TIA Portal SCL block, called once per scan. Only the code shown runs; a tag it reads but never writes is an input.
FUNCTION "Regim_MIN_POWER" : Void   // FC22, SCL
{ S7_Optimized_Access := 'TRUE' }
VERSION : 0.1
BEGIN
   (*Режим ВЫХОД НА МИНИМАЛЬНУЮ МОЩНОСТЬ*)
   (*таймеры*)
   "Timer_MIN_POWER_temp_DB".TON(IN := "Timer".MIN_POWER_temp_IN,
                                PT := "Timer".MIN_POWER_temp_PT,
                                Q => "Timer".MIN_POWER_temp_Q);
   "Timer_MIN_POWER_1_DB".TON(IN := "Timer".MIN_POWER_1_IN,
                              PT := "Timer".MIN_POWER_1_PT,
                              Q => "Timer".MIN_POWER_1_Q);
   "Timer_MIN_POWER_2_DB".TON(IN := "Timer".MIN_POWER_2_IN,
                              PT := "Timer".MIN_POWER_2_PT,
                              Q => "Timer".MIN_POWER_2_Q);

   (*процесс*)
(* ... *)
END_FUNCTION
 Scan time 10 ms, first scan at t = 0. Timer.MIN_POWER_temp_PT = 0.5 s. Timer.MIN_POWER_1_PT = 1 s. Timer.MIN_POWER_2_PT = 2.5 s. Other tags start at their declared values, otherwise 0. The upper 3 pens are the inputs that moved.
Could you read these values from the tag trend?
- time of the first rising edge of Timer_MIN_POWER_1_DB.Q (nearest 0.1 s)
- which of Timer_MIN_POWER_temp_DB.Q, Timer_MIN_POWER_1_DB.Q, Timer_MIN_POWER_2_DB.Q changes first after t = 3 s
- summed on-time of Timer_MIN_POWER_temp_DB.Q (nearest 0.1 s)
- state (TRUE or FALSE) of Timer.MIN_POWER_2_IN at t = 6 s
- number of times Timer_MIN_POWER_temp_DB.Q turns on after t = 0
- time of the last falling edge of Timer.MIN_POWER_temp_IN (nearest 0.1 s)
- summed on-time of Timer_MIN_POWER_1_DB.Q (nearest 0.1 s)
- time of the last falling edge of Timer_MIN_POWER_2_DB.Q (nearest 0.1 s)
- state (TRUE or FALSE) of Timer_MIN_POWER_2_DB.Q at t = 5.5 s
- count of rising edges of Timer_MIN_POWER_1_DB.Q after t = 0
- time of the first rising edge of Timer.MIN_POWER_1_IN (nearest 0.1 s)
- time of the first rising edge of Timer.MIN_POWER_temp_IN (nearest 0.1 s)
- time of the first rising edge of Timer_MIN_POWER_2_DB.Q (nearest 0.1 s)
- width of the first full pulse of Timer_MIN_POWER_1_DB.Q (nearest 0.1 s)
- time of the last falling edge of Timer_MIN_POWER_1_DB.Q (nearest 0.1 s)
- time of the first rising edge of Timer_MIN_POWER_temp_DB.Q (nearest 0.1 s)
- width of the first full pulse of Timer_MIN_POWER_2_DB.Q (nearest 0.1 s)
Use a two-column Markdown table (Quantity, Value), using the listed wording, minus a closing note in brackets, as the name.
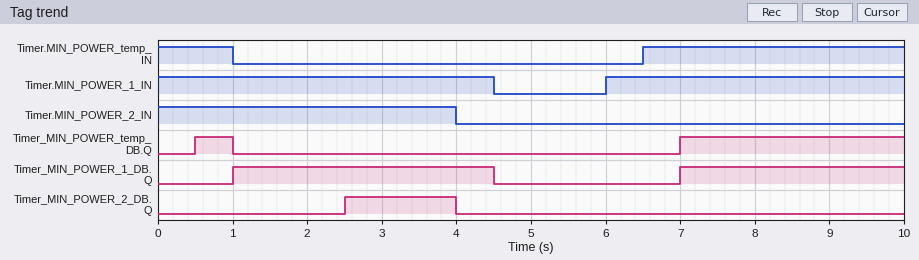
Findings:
| Quantity | Value |
|---|---|
| time of the first rising edge of Timer_MIN_POWER_1_DB.Q | 1.0 s |
| which of Timer_MIN_POWER_temp_DB.Q, Timer_MIN_POWER_1_DB.Q, Timer_MIN_POWER_2_DB.Q changes first after t = 3 s | Timer_MIN_POWER_2_DB.Q |
| summed on-time of Timer_MIN_POWER_temp_DB.Q | 3.5 s |
| state (TRUE or FALSE) of Timer.MIN_POWER_2_IN at t = 6 s | FALSE |
| number of times Timer_MIN_POWER_temp_DB.Q turns on after t = 0 | 2 |
| time of the last falling edge of Timer.MIN_POWER_temp_IN | 1.0 s |
| summed on-time of Timer_MIN_POWER_1_DB.Q | 6.5 s |
| time of the last falling edge of Timer_MIN_POWER_2_DB.Q | 4.0 s |
| state (TRUE or FALSE) of Timer_MIN_POWER_2_DB.Q at t = 5.5 s | FALSE |
| count of rising edges of Timer_MIN_POWER_1_DB.Q after t = 0 | 2 |
| time of the first rising edge of Timer.MIN_POWER_1_IN | 6.0 s |
| time of the first rising edge of Timer.MIN_POWER_temp_IN | 6.5 s |
| time of the first rising edge of Timer_MIN_POWER_2_DB.Q | 2.5 s |
| width of the first full pulse of Timer_MIN_POWER_1_DB.Q | 3.5 s |
| time of the last falling edge of Timer_MIN_POWER_1_DB.Q | 4.5 s |
| time of the first rising edge of Timer_MIN_POWER_temp_DB.Q | 0.5 s |
| width of the first full pulse of Timer_MIN_POWER_2_DB.Q | 1.5 s |
